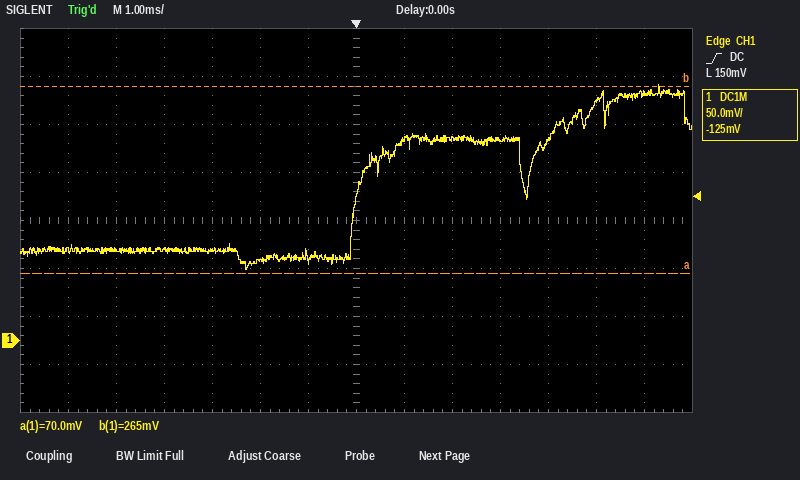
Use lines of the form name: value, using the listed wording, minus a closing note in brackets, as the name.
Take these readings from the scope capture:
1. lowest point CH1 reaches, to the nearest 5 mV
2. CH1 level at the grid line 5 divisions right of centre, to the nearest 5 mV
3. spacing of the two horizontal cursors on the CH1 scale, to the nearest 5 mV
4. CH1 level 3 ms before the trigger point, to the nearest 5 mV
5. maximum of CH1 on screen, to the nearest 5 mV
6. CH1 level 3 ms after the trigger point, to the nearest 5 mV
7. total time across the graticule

lowest point CH1 reaches, to the nearest 5 mV: 75 mV
CH1 level at the grid line 5 divisions right of centre, to the nearest 5 mV: 250 mV
spacing of the two horizontal cursors on the CH1 scale, to the nearest 5 mV: 195 mV
CH1 level 3 ms before the trigger point, to the nearest 5 mV: 95 mV
maximum of CH1 on screen, to the nearest 5 mV: 265 mV
CH1 level 3 ms after the trigger point, to the nearest 5 mV: 210 mV
total time across the graticule: 14 ms
